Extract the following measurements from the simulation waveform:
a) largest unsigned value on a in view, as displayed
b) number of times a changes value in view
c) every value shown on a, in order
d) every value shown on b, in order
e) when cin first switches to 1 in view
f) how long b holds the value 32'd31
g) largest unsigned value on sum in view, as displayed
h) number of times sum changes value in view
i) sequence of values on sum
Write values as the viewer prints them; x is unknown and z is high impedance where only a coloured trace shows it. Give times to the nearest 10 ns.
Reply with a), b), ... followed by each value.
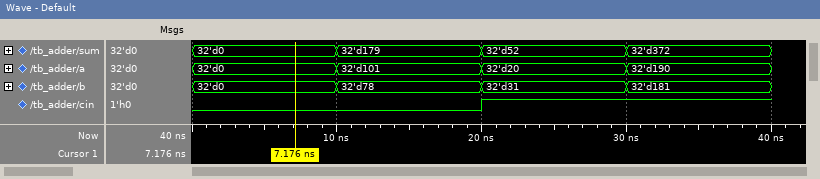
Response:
a) 32'd190
b) 3
c) 32'd0, 32'd101, 32'd20, 32'd190
d) 32'd0, 32'd78, 32'd31, 32'd181
e) 20 ns
f) 10 ns
g) 32'd372
h) 3
i) 32'd0, 32'd179, 32'd52, 32'd372
